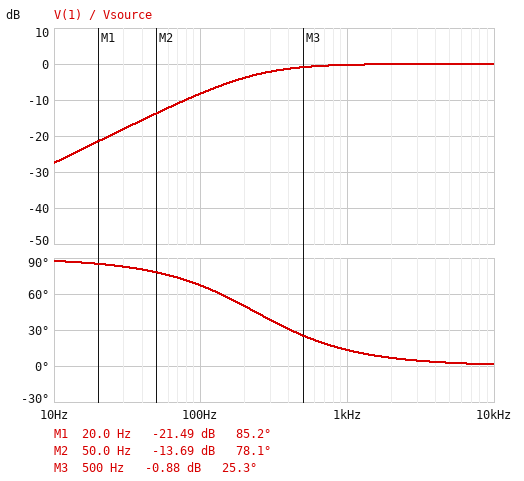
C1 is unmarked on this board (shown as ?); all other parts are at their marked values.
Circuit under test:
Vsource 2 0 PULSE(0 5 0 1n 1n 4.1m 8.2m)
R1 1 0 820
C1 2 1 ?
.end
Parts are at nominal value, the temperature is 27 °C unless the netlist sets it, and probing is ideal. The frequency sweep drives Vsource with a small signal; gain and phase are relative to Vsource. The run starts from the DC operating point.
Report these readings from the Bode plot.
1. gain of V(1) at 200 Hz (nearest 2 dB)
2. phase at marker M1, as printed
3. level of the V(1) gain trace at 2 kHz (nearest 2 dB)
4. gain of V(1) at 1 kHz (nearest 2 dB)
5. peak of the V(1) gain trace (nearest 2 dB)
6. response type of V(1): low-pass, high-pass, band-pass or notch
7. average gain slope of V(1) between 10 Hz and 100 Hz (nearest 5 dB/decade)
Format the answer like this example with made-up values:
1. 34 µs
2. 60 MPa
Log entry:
1. -4 dB
2. 85.2 deg
3. 0 dB
4. 0 dB
5. 0 dB
6. high-pass
7. 20 dB/decade
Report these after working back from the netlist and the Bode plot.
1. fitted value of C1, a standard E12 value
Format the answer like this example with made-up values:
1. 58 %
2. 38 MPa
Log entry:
1. 820 nF
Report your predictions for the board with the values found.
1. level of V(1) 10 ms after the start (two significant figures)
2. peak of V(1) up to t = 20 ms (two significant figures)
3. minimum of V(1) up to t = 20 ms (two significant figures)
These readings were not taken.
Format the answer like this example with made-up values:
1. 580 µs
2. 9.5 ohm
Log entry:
1. 340 mV
2. 5.0 V
3. -5.0 V
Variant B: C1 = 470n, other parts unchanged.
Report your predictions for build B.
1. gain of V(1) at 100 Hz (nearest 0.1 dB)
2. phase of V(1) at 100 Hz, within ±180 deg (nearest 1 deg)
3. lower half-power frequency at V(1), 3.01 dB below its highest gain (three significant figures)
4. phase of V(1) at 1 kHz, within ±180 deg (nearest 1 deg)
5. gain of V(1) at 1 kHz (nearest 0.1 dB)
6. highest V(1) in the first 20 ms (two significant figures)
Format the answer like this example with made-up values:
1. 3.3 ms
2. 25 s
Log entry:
1. -12.6 dB
2. 76 deg
3. 413 Hz
4. 22 deg
5. -0.7 dB
6. 5.0 V
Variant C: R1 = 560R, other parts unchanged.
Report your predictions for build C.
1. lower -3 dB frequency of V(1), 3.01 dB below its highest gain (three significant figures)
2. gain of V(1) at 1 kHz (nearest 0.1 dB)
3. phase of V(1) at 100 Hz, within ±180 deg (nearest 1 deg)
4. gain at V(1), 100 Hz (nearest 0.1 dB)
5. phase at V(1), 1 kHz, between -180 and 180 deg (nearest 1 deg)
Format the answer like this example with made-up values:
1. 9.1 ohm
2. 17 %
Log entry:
1. 347 Hz
2. -0.5 dB
3. 74 deg
4. -11.1 dB
5. 19 deg
